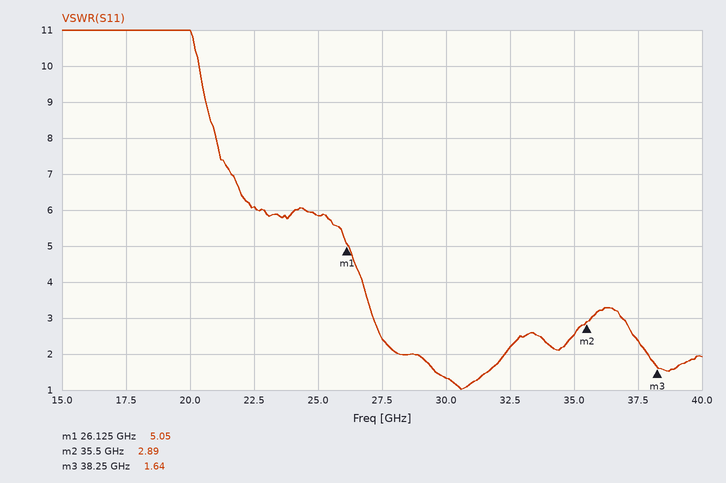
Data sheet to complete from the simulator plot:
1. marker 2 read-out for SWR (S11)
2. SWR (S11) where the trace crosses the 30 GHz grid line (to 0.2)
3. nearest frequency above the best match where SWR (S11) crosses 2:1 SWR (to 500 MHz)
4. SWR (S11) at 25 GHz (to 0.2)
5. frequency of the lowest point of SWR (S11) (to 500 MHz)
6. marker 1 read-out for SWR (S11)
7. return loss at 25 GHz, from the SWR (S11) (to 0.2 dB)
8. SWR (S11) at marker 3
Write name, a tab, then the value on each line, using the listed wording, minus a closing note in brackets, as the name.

marker 2 read-out for SWR	2.89
SWR (S11) where the trace crosses the 30 GHz grid line	1.4
nearest frequency above the best match where SWR (S11) crosses 2:1 SWR	32.5 GHz
SWR (S11) at 25 GHz	5.8
frequency of the lowest point of SWR (S11)	30.5 GHz
marker 1 read-out for SWR	5.05
return loss at 25 GHz, from the SWR (S11)	3.0 dB
SWR (S11) at marker 3	1.64
